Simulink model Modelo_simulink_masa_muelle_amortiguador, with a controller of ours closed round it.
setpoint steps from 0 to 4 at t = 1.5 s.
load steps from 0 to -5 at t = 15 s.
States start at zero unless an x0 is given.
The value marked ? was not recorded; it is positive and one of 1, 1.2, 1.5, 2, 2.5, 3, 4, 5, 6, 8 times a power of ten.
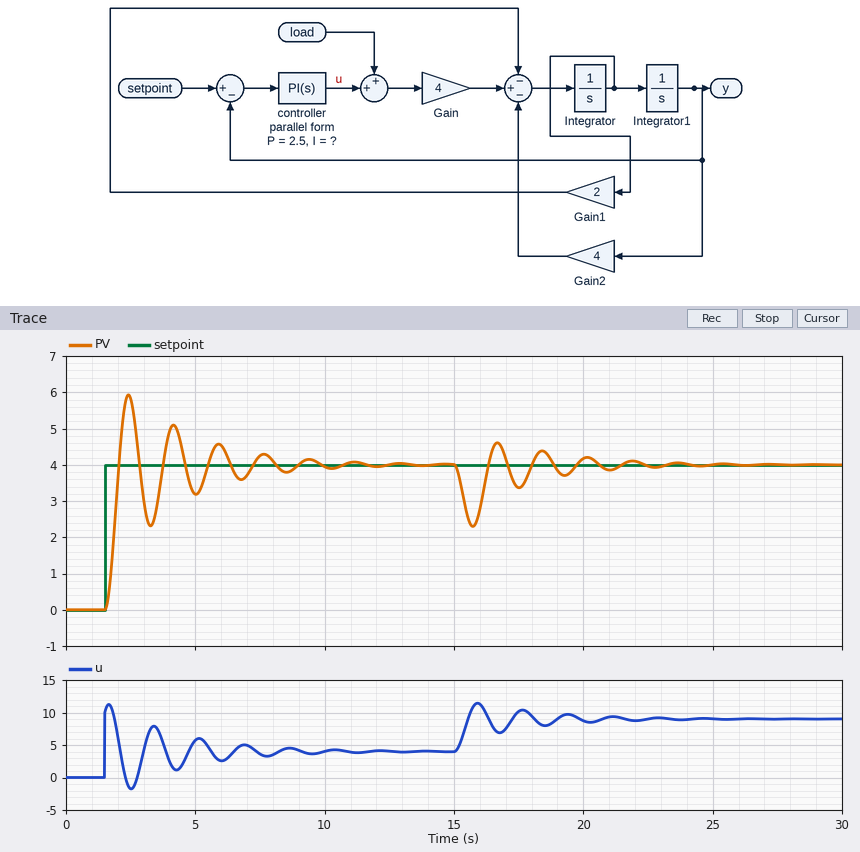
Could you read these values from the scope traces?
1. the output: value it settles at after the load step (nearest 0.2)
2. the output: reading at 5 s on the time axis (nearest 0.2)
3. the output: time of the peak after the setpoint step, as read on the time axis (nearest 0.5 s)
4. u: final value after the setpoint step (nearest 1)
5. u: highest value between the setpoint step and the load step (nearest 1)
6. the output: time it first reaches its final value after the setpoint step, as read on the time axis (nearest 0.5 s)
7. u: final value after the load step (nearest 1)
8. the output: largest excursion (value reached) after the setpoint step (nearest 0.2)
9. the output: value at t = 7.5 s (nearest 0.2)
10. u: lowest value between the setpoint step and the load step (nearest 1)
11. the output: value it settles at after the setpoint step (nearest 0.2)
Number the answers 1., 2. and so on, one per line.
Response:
1. 4.0
2. 3.2
3. 2.5 s
4. 4
5. 11
6. 2.0 s
7. 9
8. 6.0
9. 4.2
10. -2
11. 4.0
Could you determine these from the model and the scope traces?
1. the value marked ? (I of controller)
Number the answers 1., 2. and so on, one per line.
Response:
1. 4
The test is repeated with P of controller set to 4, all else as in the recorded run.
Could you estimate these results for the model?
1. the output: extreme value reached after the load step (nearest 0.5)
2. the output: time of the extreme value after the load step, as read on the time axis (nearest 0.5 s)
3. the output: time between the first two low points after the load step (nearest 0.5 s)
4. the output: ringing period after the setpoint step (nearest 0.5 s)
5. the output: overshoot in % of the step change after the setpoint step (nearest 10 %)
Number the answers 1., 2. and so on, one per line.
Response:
1. 2.5
2. 15.5 s
3. 1.5 s
4. 1.5 s
5. 50 %
